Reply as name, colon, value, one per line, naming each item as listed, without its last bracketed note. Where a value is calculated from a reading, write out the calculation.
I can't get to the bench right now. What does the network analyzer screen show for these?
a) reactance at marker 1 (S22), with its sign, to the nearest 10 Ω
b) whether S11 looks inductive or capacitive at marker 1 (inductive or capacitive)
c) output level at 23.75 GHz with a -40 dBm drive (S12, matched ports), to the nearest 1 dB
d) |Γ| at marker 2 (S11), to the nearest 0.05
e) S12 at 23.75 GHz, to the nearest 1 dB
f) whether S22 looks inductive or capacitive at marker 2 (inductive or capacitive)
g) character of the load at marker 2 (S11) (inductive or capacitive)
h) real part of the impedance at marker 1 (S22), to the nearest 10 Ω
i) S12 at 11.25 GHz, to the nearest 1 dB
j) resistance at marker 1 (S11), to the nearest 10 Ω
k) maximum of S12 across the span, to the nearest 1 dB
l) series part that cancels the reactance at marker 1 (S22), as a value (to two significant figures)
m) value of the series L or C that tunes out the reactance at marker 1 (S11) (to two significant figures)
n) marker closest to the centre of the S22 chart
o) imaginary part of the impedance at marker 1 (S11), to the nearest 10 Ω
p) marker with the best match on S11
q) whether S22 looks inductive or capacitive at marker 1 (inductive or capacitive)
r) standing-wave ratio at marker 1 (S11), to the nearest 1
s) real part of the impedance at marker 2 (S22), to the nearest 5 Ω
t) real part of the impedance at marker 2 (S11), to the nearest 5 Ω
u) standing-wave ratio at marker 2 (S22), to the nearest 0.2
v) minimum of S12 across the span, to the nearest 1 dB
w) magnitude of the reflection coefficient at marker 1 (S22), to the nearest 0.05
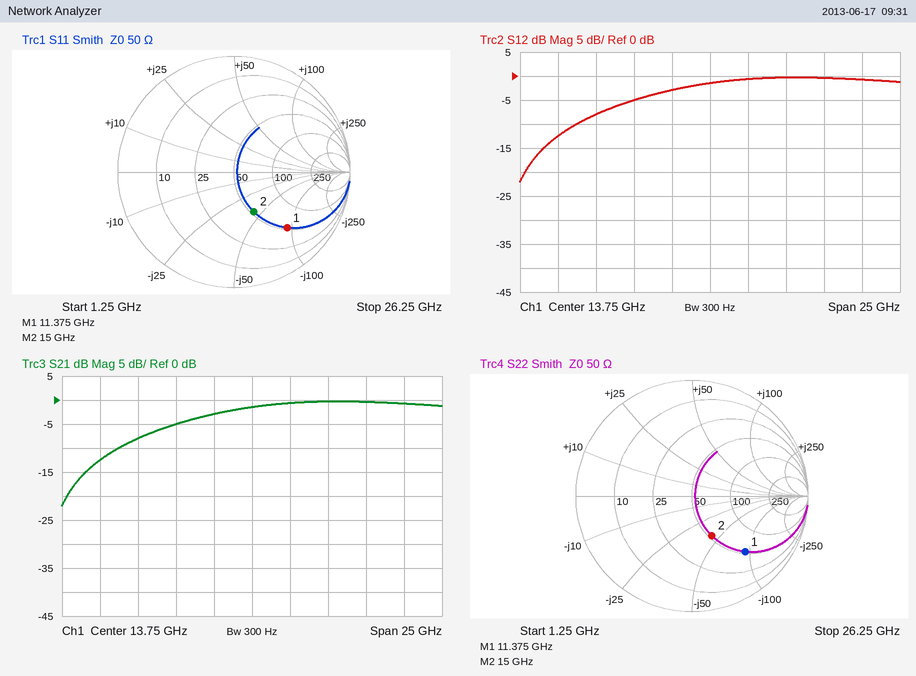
reactance at marker 1 (S22), with its sign, to the nearest 10 Ω: -90 Ω
whether S11 looks inductive or capacitive at marker 1: capacitive
output level at 23.75 GHz with a -40 dBm drive (S12, matched ports), to the nearest 1 dB: -40 dBm + (-1 dB) = -41 dBm
|Γ| at marker 2 (S11), to the nearest 0.05: 0.40
S12 at 23.75 GHz, to the nearest 1 dB: -1 dB
whether S22 looks inductive or capacitive at marker 2: capacitive
character of the load at marker 2 (S11): capacitive
real part of the impedance at marker 1 (S22), to the nearest 10 Ω: 50 Ω
S12 at 11.25 GHz, to the nearest 1 dB: -3 dB
resistance at marker 1 (S11), to the nearest 10 Ω: 50 Ω
maximum of S12 across the span, to the nearest 1 dB: 0 dB
series part that cancels the reactance at marker 1 (S22), as a value: L = 90 Ω/(2π × 11.375 GHz) ≈ 1.3 nH
value of the series L or C that tunes out the reactance at marker 1 (S11): L = 90 Ω/(2π × 11.375 GHz) ≈ 1.3 nH
marker closest to the centre of the S22 chart: marker 2
imaginary part of the impedance at marker 1 (S11), to the nearest 10 Ω: -90 Ω
marker with the best match on S11: marker 2
whether S22 looks inductive or capacitive at marker 1: capacitive
standing-wave ratio at marker 1 (S11), to the nearest 1: 5
real part of the impedance at marker 2 (S22), to the nearest 5 Ω: 55 Ω
real part of the impedance at marker 2 (S11), to the nearest 5 Ω: 55 Ω
standing-wave ratio at marker 2 (S22), to the nearest 0.2: 2.2
minimum of S12 across the span, to the nearest 1 dB: -22 dB
magnitude of the reflection coefficient at marker 1 (S22), to the nearest 0.05: 0.65
